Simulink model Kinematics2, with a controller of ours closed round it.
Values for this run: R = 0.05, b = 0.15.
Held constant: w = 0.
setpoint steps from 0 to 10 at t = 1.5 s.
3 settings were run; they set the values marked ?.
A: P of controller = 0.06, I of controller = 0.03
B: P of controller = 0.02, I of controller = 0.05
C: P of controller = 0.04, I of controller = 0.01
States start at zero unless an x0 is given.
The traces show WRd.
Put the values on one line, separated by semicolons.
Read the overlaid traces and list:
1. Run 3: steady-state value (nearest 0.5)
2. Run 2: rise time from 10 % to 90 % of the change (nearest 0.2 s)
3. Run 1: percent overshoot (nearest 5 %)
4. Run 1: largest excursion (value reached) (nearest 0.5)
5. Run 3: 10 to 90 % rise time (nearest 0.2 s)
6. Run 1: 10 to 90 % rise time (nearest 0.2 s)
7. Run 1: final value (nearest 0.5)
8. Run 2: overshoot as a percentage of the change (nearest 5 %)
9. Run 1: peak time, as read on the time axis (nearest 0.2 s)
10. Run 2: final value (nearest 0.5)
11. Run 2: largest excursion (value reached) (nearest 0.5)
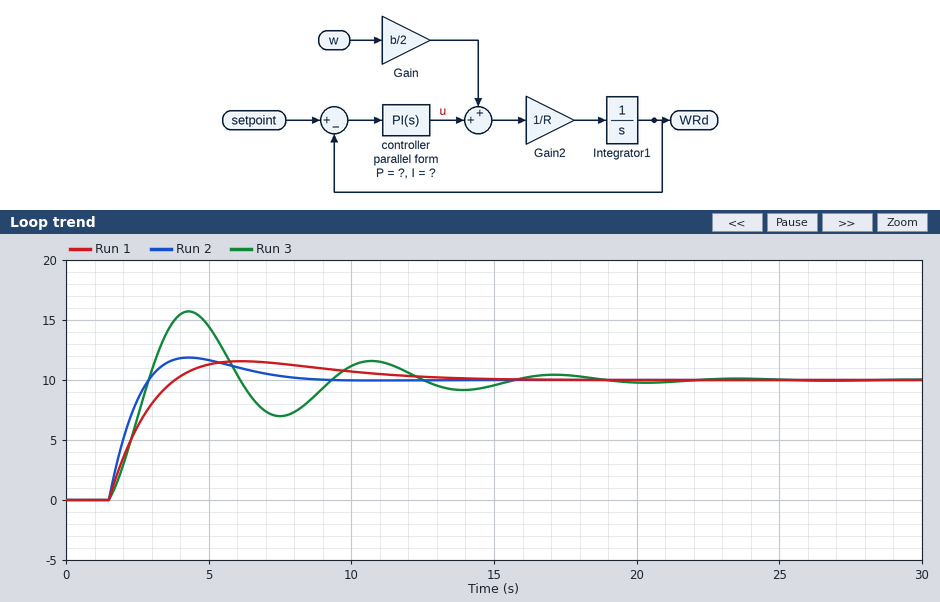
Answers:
10.0; 1.0 s; 15 %; 11.5; 1.0 s; 1.8 s; 10.0; 20 %; 6.2 s; 10.0; 12.0
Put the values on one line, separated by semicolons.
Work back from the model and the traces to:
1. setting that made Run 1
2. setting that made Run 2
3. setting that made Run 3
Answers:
C; A; B
